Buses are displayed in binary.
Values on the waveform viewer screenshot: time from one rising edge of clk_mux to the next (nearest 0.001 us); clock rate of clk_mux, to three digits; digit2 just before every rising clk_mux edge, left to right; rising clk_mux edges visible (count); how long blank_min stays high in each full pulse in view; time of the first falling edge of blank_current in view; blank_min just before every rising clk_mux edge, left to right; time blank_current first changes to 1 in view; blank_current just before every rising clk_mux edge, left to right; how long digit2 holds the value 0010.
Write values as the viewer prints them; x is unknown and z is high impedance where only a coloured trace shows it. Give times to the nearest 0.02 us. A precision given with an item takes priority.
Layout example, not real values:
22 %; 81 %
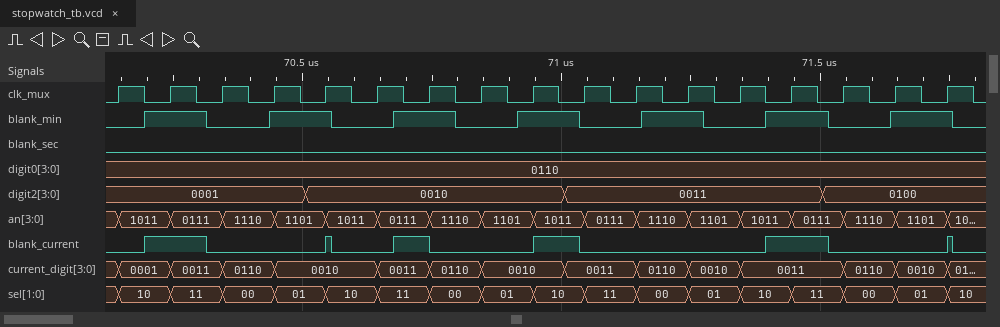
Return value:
0.1 us; 10.0 MHz; 0001, 0001, 0001, 0001, 0010, 0010, 0010, 0010, 0010, 0011, 0011, 0011, 0011, 0011, 0100, 0100, 0100; 17; 0.12 us, 0.12 us, 0.12 us, 0.12 us, 0.12 us, 0.12 us, 0.12 us; 70.32 us; 0 1 0 1 1 0 1 0 1 0 0 1 0 1 0 1 1; 70.2 us; 0 1 0 0 0 0 1 0 0 0 0 0 0 1 0 0 0; 0.5 us
